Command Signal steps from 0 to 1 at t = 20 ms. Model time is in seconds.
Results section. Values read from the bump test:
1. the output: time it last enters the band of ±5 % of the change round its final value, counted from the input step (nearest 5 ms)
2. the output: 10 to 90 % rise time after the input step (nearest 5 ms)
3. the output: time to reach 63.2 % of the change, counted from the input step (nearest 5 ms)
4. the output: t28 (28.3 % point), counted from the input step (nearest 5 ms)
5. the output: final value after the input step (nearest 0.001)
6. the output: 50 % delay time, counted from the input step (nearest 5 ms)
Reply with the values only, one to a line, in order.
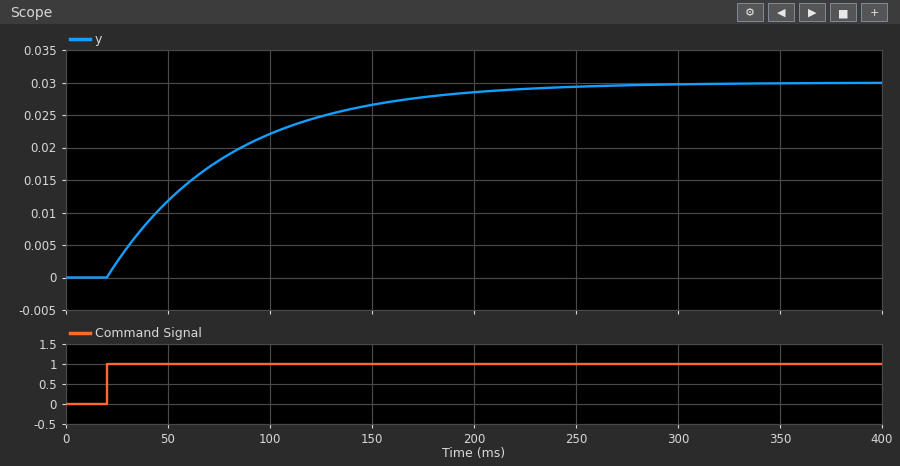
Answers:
180 ms
130 ms
60 ms
20 ms
0.030
40 ms
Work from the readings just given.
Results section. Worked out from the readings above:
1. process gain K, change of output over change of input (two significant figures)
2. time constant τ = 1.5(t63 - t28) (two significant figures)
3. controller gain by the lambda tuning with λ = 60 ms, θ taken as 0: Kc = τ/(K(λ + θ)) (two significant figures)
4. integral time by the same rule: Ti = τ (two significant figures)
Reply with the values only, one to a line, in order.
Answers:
0.030
60 ms
33
60 ms
